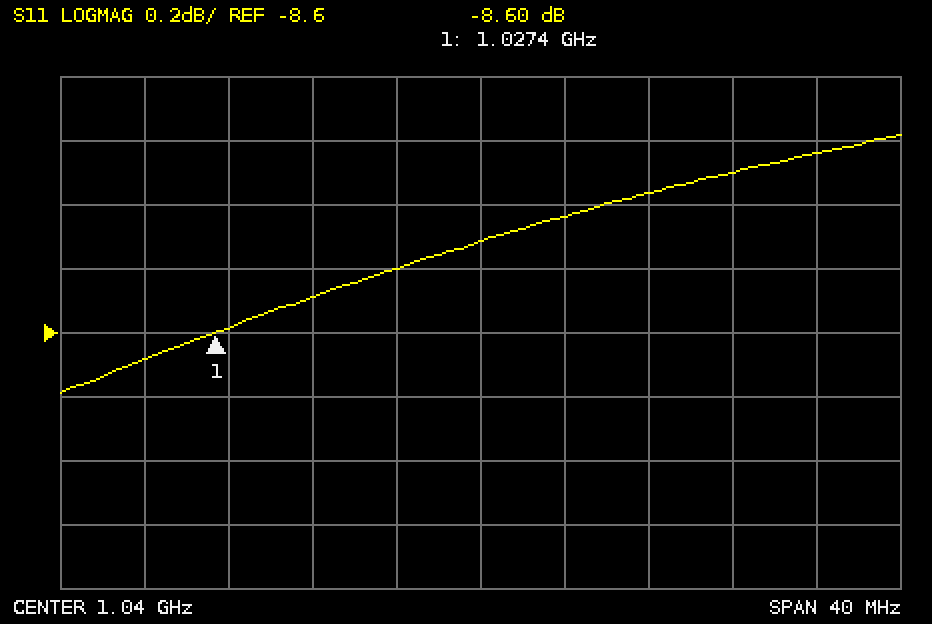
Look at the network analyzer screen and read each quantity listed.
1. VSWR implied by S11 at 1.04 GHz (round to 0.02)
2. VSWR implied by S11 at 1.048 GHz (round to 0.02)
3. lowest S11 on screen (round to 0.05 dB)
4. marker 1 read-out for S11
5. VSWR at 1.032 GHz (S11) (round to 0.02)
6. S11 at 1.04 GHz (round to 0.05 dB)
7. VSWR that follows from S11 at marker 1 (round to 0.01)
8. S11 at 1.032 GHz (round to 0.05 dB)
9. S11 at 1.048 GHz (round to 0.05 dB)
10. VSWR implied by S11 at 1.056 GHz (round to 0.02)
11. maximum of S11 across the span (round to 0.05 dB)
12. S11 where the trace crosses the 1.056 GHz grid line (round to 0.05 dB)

2.24
2.28
-8.80 dB
-8.60 dB
2.20
-8.30 dB
2.18
-8.50 dB
-8.15 dB
2.32
-8.00 dB
-8.05 dB
